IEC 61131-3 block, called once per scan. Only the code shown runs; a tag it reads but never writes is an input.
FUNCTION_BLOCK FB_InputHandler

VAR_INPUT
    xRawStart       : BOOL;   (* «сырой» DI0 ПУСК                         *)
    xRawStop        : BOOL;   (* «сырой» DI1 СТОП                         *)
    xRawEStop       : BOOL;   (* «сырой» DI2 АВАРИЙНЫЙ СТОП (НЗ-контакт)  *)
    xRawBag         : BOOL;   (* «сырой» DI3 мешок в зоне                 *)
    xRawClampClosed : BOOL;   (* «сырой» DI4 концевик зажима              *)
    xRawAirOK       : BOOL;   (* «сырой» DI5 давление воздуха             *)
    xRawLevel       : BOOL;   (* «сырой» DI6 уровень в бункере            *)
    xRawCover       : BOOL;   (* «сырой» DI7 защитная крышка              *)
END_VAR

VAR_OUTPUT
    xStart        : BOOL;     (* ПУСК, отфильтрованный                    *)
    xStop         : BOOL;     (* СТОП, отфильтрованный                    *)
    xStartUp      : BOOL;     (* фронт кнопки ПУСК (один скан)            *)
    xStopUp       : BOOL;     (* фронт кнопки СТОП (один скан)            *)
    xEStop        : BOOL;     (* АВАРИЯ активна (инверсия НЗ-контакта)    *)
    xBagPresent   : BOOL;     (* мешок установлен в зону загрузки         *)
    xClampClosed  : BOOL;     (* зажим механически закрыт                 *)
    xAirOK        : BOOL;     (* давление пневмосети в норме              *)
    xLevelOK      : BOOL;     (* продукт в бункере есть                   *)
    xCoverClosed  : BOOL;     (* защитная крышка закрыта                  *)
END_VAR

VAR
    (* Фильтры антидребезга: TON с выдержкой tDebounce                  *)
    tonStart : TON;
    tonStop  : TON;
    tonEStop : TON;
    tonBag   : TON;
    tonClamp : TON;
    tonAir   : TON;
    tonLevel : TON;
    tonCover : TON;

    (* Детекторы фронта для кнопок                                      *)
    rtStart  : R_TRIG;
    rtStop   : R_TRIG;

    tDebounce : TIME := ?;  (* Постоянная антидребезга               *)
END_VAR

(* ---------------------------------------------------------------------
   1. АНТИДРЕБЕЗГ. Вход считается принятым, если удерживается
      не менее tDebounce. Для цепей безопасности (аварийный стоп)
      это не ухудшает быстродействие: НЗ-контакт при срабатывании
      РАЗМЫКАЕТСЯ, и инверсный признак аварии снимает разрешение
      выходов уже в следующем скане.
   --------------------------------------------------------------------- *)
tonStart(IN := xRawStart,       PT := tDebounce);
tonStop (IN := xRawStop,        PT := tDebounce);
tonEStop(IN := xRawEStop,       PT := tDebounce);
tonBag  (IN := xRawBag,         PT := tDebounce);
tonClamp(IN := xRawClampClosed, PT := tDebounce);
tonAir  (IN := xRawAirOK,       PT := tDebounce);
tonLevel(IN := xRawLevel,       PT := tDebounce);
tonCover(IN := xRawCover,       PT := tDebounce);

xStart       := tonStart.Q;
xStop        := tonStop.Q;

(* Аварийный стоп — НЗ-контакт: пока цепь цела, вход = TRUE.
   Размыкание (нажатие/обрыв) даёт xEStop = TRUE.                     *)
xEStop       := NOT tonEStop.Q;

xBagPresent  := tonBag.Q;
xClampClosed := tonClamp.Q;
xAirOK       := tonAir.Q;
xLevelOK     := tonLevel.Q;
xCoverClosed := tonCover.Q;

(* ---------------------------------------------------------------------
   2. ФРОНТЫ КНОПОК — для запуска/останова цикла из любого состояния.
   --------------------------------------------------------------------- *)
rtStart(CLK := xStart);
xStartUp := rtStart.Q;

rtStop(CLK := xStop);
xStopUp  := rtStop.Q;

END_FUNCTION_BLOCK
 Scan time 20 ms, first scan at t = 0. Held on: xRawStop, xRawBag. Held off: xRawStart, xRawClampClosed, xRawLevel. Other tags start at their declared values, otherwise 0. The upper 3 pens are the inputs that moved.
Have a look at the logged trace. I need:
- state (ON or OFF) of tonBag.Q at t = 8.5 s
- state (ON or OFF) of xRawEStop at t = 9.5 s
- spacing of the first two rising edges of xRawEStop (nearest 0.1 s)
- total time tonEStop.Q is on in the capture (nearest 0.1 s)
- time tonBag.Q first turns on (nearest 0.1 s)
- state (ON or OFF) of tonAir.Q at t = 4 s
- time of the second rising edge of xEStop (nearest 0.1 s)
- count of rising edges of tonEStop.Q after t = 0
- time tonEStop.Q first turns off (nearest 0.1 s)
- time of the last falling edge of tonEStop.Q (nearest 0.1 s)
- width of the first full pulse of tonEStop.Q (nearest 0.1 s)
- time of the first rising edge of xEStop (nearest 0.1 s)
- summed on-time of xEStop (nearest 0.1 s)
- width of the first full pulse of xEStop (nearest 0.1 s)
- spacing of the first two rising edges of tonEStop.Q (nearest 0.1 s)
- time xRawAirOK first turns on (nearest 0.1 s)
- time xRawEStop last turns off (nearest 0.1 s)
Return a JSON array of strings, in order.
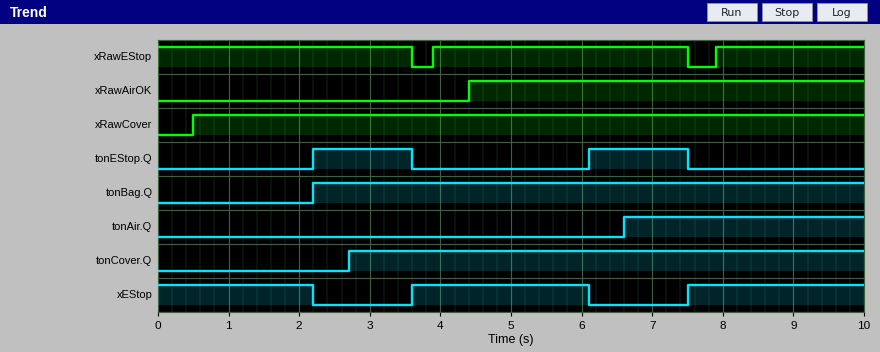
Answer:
["ON", "ON", "4.0 s", "2.8 s", "2.2 s", "OFF", "7.5 s", "2", "3.6 s", "7.5 s", "1.4 s", "3.6 s", "7.2 s", "2.5 s", "3.9 s", "4.4 s", "7.5 s"]
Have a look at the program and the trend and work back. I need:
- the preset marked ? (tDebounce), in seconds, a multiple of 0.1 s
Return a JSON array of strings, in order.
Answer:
["2.2 s"]
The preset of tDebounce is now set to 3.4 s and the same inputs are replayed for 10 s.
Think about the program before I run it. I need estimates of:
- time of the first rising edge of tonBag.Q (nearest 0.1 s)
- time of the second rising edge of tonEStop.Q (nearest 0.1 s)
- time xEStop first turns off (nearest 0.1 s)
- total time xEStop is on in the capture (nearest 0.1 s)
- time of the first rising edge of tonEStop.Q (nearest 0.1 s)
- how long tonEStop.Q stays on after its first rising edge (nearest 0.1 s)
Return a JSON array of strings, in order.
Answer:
["3.4 s", "7.3 s", "3.4 s", "9.6 s", "3.4 s", "0.2 s"]
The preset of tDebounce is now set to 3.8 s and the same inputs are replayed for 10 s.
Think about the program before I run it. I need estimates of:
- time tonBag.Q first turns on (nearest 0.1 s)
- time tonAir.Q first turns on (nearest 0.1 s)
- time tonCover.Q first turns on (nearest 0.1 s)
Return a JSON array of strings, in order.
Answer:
["3.8 s", "8.2 s", "4.3 s"]
